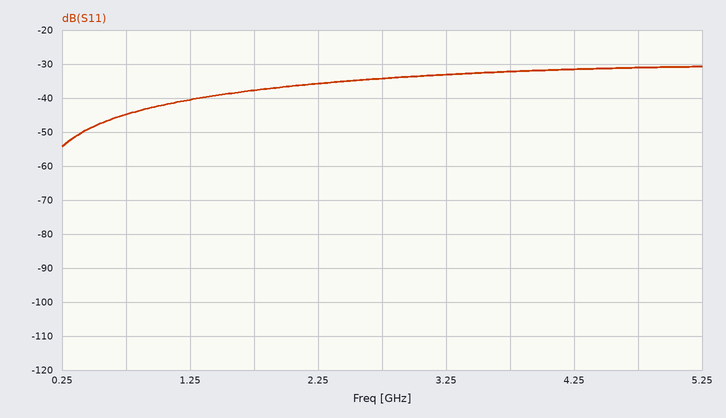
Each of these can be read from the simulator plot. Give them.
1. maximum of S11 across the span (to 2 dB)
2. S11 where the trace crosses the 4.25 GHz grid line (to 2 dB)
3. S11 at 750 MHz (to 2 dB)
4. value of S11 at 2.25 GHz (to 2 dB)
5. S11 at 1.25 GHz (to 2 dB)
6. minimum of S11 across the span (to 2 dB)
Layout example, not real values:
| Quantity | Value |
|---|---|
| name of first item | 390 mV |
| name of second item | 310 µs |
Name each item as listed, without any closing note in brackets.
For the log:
| Quantity | Value |
|---|---|
| maximum of S11 across the span | -30 dB |
| S11 where the trace crosses the 4.25 GHz grid line | -32 dB |
| S11 at 750 MHz | -44 dB |
| value of S11 at 2.25 GHz | -36 dB |
| S11 at 1.25 GHz | -40 dB |
| minimum of S11 across the span | -54 dB |
